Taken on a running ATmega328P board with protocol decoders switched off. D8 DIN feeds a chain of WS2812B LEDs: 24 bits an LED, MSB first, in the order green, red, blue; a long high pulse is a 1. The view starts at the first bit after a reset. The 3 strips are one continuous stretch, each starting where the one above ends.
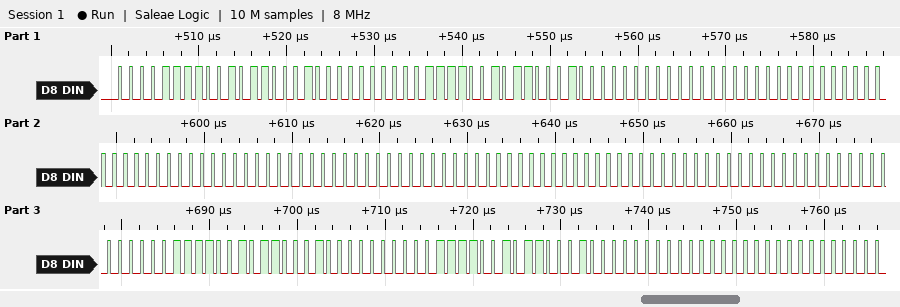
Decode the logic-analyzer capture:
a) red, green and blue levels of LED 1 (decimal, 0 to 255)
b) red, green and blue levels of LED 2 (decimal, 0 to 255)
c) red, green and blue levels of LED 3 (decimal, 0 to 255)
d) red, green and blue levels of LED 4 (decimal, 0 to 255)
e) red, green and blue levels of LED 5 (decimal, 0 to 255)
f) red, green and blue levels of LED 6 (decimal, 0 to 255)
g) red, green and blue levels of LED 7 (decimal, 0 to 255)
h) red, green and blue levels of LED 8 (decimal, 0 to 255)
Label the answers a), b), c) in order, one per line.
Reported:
a) 44, 15, 64
b) 44, 15, 64
c) 0, 0, 0
d) 0, 0, 0
e) 0, 0, 0
f) 0, 0, 0
g) 44, 15, 64
h) 44, 15, 64
